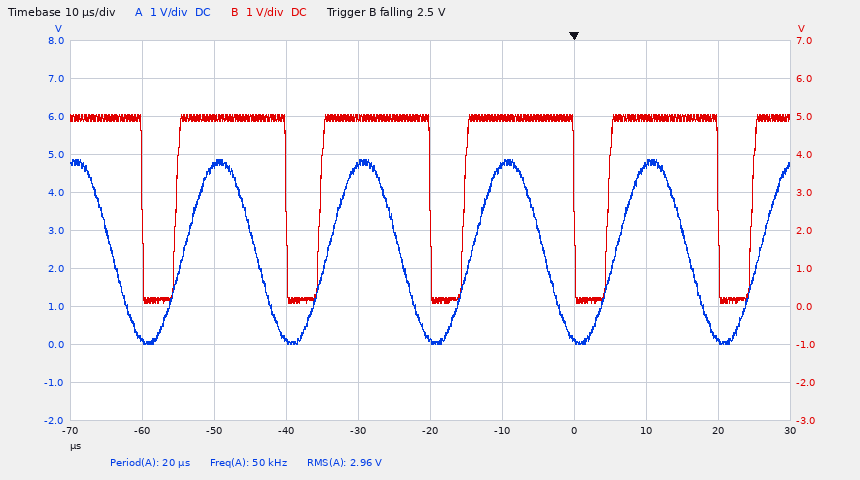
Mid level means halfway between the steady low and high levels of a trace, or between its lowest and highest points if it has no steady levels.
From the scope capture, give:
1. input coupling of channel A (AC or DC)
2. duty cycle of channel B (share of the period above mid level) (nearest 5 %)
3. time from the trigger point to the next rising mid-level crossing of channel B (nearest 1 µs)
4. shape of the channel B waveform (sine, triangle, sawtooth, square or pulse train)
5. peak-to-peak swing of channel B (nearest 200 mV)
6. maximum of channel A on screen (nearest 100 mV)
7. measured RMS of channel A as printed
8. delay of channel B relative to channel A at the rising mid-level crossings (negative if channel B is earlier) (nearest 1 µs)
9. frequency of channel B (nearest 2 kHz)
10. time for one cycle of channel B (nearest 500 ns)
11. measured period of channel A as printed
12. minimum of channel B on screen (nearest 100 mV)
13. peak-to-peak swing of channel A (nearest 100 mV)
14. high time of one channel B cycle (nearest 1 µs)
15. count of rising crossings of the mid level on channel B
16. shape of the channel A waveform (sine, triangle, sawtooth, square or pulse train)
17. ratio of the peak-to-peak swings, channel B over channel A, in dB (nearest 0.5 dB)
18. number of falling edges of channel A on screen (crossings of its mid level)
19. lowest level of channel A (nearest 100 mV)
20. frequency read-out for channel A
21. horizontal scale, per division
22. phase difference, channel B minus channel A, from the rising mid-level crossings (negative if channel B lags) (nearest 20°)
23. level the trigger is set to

DC
75 %
5 µs
pulse train
5.0 V
4.9 V
2.96 V
-1 µs
50 kHz
20.0 µs
20 µs
100 mV
4.9 V
15 µs
5
sine
0.0 dB
5
0.0 V
50 kHz
10 µs
+20°
2.5 V
